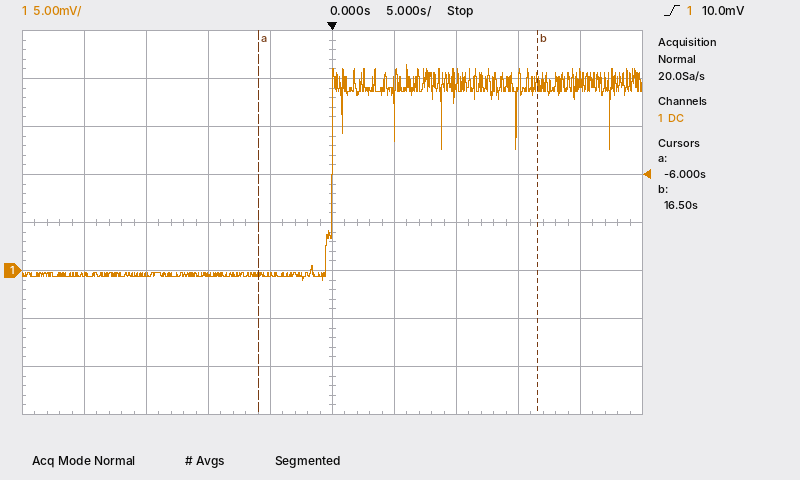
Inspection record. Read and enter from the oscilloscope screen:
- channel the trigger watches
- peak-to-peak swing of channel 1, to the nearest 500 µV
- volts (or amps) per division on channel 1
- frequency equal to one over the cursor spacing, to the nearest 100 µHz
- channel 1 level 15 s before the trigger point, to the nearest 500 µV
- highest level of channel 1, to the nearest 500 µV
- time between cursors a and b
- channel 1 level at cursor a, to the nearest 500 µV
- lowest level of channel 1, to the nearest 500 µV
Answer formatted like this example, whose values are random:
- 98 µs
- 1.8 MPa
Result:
- channel 1
- 22.5 mV
- 5 mV
- 44.4 mHz
- -500 µV
- 21.5 mV
- 22.5 s
- -500 µV
- -1.0 mV
